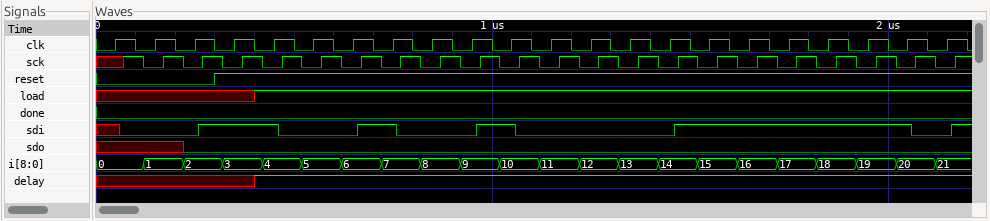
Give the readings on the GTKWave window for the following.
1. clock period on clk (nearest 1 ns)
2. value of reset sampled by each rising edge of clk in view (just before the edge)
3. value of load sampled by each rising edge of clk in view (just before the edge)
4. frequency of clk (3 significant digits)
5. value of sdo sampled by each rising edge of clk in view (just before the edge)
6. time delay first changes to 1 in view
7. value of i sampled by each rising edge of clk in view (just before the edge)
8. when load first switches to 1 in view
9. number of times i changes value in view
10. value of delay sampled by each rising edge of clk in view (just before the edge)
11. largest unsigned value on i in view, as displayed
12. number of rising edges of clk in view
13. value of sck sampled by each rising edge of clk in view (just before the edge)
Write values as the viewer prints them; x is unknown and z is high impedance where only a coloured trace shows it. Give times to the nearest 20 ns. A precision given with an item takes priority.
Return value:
100 ns
0 0 0 1 1 1 1 1 1 1 1 1 1 1 1 1 1 1 1 1 1 1
x x x x 1 1 1 1 1 1 1 1 1 1 1 1 1 1 1 1 1 1
10.0 MHz
x x 0 0 0 0 0 0 0 0 0 0 0 0 0 0 0 0 0 0 0 0
400 ns
0, 1, 2, 3, 4, 5, 6, 7, 8, 9, 10, 11, 12, 13, 14, 15, 16, 17, 18, 19, 20, 21
400 ns
21
x x x x 1 1 1 1 1 1 1 1 1 1 1 1 1 1 1 1 1 1
21
22
x 0 0 0 0 0 0 0 0 0 0 0 0 0 0 0 0 0 0 0 0 0
